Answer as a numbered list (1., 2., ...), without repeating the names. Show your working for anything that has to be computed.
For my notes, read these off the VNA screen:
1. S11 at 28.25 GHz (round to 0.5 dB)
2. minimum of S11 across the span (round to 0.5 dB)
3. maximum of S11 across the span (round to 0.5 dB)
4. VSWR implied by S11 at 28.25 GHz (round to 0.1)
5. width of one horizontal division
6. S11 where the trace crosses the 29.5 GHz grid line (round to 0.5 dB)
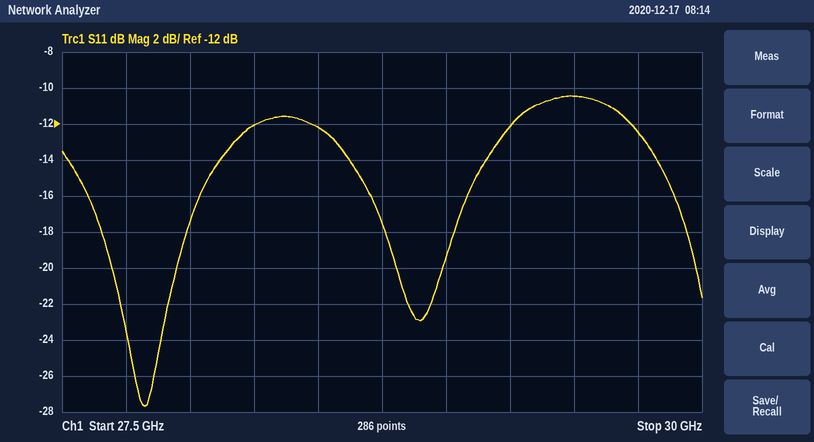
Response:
1. -12.0 dB
2. -27.5 dB
3. -10.5 dB
4. |Γ| = 10^(-12/20) = 0.2512; VSWR = (1 + 0.2512)/(1 − 0.2512) ≈ 1.7
5. 250 MHz
6. -10.5 dB
